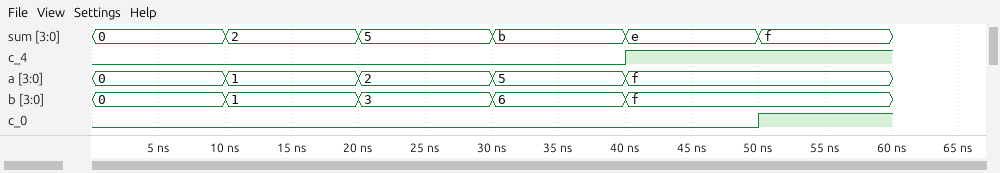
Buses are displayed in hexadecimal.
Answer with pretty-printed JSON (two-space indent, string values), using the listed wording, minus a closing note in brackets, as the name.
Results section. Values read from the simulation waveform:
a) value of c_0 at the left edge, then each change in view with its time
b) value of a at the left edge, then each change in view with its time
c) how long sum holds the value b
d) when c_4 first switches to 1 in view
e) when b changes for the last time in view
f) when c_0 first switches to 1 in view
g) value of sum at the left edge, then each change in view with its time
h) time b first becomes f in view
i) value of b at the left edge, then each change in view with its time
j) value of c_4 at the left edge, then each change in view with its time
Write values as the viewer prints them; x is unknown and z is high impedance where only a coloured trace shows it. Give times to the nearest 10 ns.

{
  "value of c_0 at the left edge, then each change in view with its time": "0, 1 at 50 ns",
  "value of a at the left edge, then each change in view with its time": "0, 1 at 10 ns, 2 at 20 ns, 5 at 30 ns, f at 40 ns",
  "how long sum holds the value b": "10 ns",
  "when c_4 first switches to 1 in view": "40 ns",
  "when b changes for the last time in view": "40 ns",
  "when c_0 first switches to 1 in view": "50 ns",
  "value of sum at the left edge, then each change in view with its time": "0, 2 at 10 ns, 5 at 20 ns, b at 30 ns, e at 40 ns, f at 50 ns",
  "time b first becomes f in view": "40 ns",
  "value of b at the left edge, then each change in view with its time": "0, 1 at 10 ns, 3 at 20 ns, 6 at 30 ns, f at 40 ns",
  "value of c_4 at the left edge, then each change in view with its time": "0, 1 at 40 ns"
}
